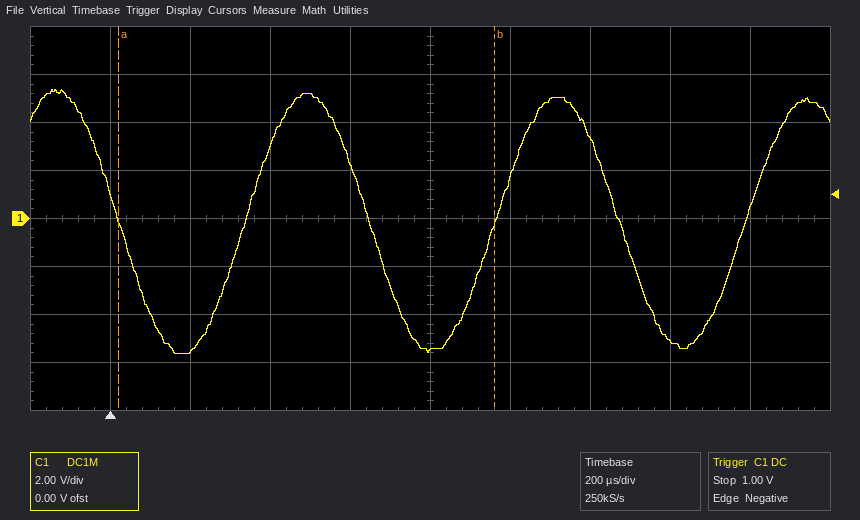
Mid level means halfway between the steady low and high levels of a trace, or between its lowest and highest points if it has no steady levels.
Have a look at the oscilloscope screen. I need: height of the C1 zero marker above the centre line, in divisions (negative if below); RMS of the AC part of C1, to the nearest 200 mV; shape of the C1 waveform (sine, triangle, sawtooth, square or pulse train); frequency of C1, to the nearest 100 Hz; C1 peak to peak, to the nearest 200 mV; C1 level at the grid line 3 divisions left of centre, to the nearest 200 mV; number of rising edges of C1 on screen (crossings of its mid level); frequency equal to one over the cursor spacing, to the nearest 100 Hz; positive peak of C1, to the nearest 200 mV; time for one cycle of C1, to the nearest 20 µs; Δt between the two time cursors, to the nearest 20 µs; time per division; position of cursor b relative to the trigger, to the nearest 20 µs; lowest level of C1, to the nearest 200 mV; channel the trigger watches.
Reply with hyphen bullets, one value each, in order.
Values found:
- 0.0 div
- 3.8 V
- sine
- 1.6 kHz
- 11.0 V
- -5.6 V
- 3
- 1.1 kHz
- 5.4 V
- 620 µs
- 940 µs
- 200 µs
- +960 µs
- -5.6 V
- C1
